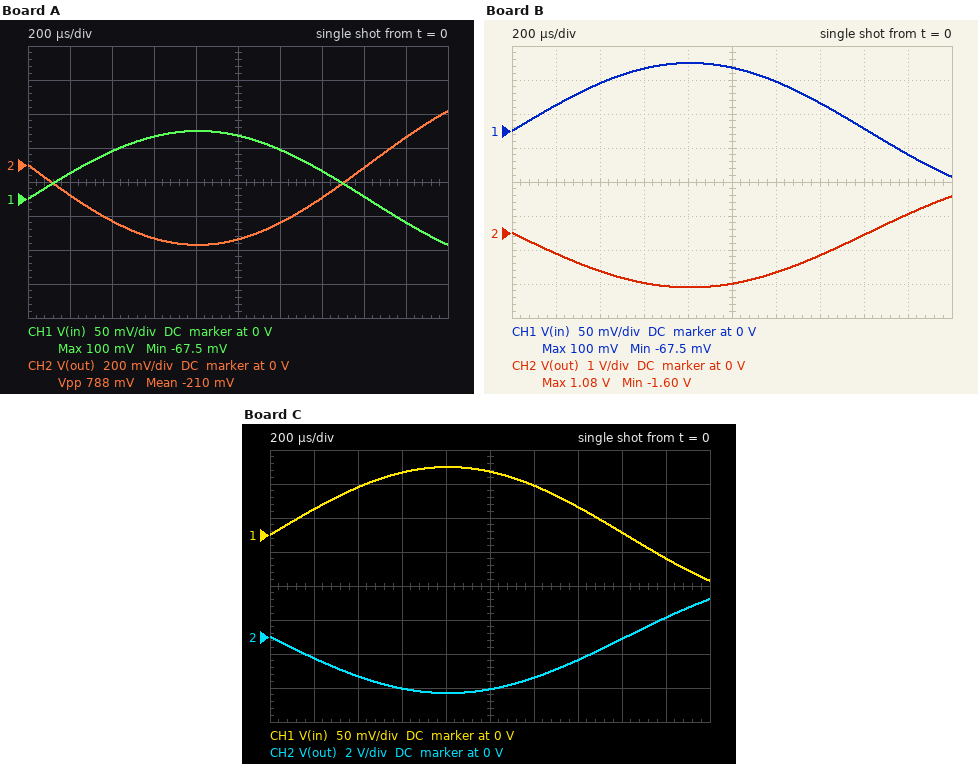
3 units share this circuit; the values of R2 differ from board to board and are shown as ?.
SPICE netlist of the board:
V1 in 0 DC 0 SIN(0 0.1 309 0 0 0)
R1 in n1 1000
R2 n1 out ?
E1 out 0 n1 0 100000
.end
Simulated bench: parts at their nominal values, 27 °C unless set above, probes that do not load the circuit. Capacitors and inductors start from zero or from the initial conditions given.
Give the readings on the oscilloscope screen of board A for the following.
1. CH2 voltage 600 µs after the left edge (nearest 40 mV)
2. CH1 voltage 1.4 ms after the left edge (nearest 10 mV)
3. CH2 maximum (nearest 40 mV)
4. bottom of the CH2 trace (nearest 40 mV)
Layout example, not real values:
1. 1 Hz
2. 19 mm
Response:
1. -440 mV
2. 40 mV
3. 320 mV
4. -480 mV
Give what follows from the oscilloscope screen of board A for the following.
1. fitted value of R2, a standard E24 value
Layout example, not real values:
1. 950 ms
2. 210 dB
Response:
1. 4.7 kΩ
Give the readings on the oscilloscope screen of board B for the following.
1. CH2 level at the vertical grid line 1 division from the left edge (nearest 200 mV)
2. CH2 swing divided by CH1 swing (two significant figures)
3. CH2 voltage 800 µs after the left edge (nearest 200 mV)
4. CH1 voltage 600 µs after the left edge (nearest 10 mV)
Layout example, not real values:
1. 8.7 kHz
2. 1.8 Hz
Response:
1. -600 mV
2. 16
3. -1.6 V
4. 90 mV
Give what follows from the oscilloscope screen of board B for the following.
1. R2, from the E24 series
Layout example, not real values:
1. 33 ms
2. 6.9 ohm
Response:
1. 16 kΩ
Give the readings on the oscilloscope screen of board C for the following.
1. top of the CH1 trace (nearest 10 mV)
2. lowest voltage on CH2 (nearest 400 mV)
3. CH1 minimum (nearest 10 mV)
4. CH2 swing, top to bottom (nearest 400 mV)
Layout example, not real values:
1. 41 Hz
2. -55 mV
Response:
1. 100 mV
2. -3.2 V
3. -70 mV
4. 5.6 V
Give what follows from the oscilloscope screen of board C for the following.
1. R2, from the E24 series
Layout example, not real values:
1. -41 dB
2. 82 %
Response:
1. 33 kΩ
